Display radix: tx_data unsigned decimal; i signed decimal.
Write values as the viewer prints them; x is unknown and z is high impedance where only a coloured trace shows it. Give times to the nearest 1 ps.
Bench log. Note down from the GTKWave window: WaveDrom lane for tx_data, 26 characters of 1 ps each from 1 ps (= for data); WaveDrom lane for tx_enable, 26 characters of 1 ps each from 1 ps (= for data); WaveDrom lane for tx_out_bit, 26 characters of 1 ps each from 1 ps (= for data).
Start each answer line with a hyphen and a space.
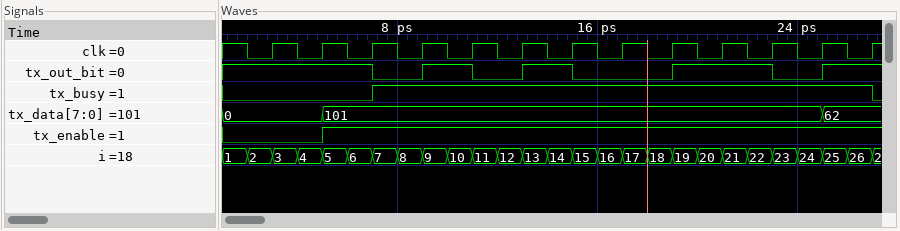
- {name: 'tx_data', wave: '=...=...................=.', data: '0 101 62'}
- {name: 'tx_enable', wave: '0...1.....................'}
- {name: 'tx_out_bit', wave: '1.....0.1.0.1.0...1...0.1.'}
